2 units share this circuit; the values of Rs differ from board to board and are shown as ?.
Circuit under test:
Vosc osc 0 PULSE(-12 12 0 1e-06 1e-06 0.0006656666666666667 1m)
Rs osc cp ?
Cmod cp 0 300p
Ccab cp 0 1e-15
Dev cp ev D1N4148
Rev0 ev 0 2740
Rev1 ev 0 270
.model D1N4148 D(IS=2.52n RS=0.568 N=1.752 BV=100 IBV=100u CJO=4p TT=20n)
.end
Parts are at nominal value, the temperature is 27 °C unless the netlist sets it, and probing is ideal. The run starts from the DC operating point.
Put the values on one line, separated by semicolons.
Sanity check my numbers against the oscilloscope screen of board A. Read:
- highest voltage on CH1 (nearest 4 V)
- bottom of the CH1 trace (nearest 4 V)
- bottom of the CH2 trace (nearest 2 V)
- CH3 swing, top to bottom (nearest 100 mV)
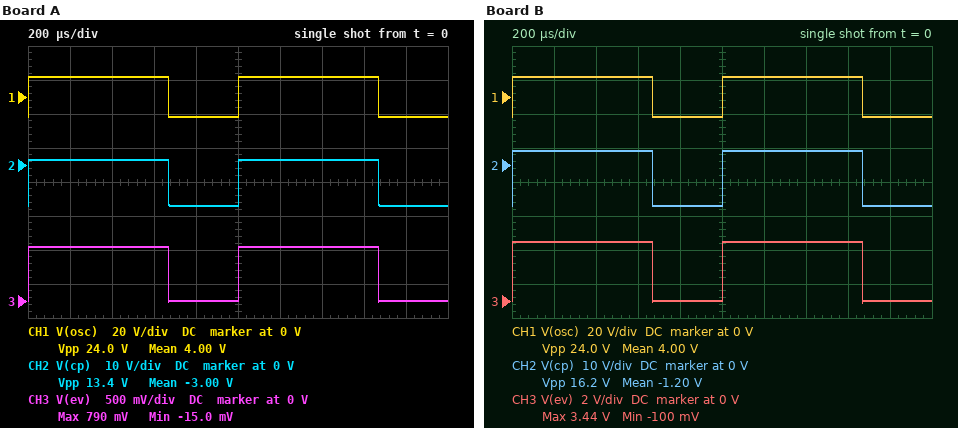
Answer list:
12 V; -12 V; -12 V; 800 mV
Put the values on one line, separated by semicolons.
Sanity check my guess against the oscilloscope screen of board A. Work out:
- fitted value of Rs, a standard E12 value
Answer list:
3.3 kΩ
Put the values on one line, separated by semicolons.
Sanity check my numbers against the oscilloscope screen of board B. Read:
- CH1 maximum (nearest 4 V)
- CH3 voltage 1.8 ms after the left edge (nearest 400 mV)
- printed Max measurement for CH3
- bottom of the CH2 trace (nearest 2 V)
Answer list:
12 V; 0 V; 3.44 V; -12 V
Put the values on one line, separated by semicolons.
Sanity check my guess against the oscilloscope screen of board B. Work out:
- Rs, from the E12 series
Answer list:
560 Ω
